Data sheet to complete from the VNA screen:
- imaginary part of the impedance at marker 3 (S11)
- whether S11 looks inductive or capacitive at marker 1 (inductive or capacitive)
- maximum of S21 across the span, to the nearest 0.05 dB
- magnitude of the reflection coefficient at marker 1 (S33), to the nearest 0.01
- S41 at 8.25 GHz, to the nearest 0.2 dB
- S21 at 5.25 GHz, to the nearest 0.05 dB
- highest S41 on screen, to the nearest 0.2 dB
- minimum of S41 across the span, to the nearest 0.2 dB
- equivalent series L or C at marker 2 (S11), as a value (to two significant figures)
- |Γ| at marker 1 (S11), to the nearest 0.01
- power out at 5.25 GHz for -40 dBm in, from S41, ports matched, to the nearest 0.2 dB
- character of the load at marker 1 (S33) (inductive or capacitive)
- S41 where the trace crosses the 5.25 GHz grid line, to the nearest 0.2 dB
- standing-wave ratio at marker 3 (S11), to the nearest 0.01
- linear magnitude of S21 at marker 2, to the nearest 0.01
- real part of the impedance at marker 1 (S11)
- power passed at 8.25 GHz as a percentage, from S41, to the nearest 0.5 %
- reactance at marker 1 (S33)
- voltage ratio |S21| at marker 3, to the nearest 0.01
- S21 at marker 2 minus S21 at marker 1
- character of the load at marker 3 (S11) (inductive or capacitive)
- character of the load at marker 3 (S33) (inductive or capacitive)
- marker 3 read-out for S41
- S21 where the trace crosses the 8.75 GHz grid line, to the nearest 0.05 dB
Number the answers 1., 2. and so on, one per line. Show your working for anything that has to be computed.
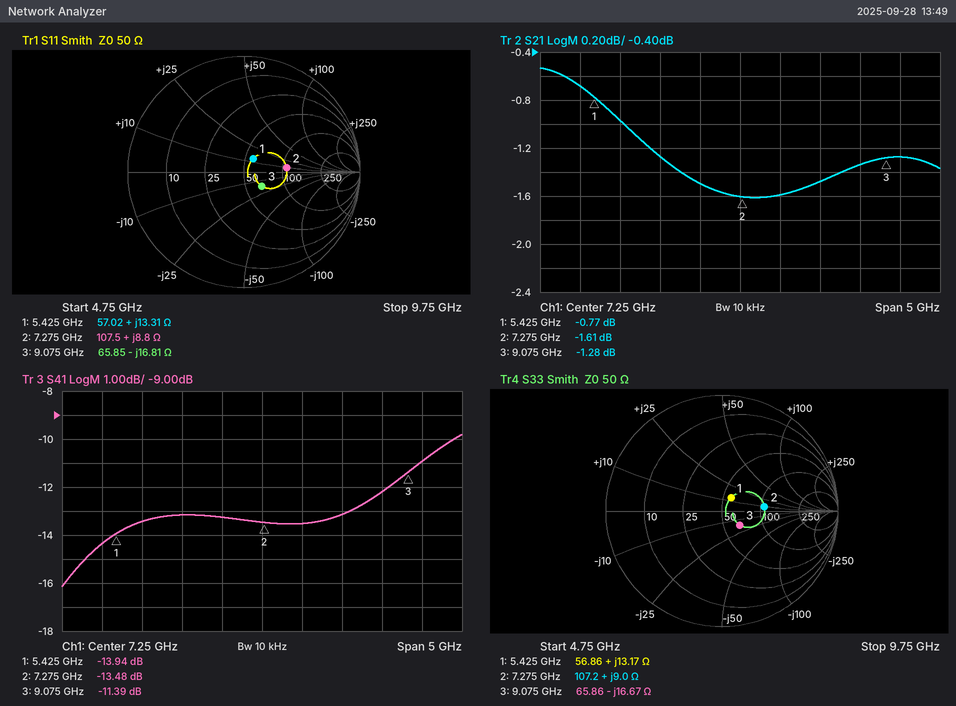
1. -16.81 Ω
2. inductive
3. -0.55 dB
4. 0.14
5. -13.2 dB
6. -0.70 dB
7. -9.8 dB
8. -16.2 dB
9. L = 8.8 Ω/(2π × 7.275 GHz) ≈ 193 pH, so 190 pH to two significant figures
10. 0.14
11. -40 dBm + (-14.4 dB) = -54.4 dBm
12. inductive
13. -14.4 dB
14. 1.49
15. 10^(-1.61/20) ≈ 0.83
16. 57.02 Ω
17. 10^(-13.2/10) ≈ 4.79 %, so 5.0 % to the nearest 0.5 %
18. +13.17 Ω
19. 10^(-1.28/20) ≈ 0.86
20. -1.61 − (-0.77) = -0.84 dB
21. capacitive
22. capacitive
23. -11.39 dB
24. -1.35 dB
